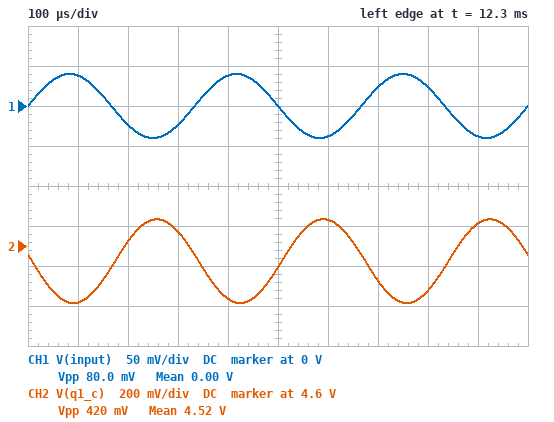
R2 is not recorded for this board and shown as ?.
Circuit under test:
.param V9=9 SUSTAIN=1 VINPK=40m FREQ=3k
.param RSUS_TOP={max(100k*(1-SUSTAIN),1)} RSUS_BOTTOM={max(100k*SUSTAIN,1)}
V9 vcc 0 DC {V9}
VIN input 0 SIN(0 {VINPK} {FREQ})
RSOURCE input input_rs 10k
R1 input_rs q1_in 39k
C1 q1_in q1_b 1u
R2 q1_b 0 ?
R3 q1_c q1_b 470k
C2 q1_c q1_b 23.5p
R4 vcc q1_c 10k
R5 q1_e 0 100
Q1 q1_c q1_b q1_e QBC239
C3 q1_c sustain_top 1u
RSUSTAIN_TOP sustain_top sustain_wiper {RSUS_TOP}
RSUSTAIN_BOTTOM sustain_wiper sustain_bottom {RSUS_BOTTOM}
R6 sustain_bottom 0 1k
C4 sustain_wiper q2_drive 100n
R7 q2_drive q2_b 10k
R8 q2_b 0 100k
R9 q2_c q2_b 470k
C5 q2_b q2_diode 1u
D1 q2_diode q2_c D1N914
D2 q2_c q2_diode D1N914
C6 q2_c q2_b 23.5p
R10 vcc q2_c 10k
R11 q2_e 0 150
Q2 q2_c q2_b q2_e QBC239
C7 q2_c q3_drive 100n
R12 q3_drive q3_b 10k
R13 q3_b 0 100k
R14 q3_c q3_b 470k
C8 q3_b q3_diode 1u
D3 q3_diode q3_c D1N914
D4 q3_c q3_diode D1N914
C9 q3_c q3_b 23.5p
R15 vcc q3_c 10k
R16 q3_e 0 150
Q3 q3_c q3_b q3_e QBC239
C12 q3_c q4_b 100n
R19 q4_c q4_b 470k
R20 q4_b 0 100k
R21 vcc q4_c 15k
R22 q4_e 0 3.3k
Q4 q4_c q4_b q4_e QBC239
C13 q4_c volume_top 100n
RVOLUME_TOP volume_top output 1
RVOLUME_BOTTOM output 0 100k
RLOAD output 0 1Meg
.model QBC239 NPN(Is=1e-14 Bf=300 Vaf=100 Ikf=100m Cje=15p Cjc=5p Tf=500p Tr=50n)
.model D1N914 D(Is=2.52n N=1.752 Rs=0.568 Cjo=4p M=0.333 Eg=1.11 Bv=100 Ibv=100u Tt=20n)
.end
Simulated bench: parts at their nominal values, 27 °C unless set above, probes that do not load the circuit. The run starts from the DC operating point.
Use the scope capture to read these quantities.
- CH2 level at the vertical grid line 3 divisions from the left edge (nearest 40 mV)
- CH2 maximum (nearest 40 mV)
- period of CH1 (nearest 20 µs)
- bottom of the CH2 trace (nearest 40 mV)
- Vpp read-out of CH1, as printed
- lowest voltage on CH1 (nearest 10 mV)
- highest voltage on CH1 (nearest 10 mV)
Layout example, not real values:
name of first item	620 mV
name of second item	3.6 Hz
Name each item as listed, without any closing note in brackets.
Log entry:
CH2 level at the vertical grid line 3 divisions from the left edge	4.68 V
CH2 maximum	4.72 V
period of CH1	340 µs
bottom of the CH2 trace	4.32 V
Vpp read-out of CH1, as printed	80.0 mV
lowest voltage on CH1	-40 mV
highest voltage on CH1	40 mV
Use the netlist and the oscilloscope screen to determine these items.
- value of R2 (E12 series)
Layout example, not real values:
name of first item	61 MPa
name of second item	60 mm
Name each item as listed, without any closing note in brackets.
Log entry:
value of R2	100 kΩ
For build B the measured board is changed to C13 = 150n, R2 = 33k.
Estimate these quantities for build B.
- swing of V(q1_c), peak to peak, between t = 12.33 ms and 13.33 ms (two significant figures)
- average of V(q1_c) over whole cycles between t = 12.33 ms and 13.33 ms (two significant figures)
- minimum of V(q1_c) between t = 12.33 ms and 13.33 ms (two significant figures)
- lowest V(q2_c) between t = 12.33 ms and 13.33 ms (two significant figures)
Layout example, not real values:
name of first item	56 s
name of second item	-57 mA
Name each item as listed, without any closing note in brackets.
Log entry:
swing of V(q1_c), peak to peak, between t = 12.33 ms and 13.33 ms	120 mV
average of V(q1_c) over whole cycles between t = 12.33 ms and 13.33 ms	8.6 V
minimum of V(q1_c) between t = 12.33 ms and 13.33 ms	8.5 V
lowest V(q2_c) between t = 12.33 ms and 13.33 ms	4.3 V
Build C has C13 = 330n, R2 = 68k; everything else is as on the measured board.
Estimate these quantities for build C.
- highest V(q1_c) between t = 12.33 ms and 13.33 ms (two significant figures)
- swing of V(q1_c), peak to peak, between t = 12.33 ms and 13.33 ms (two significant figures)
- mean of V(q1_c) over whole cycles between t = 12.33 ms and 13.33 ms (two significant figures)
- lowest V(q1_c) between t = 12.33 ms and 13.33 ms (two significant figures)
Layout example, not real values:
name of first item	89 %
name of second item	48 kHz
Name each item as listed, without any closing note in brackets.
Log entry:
highest V(q1_c) between t = 12.33 ms and 13.33 ms	5.9 V
swing of V(q1_c), peak to peak, between t = 12.33 ms and 13.33 ms	390 mV
mean of V(q1_c) over whole cycles between t = 12.33 ms and 13.33 ms	5.7 V
lowest V(q1_c) between t = 12.33 ms and 13.33 ms	5.5 V
